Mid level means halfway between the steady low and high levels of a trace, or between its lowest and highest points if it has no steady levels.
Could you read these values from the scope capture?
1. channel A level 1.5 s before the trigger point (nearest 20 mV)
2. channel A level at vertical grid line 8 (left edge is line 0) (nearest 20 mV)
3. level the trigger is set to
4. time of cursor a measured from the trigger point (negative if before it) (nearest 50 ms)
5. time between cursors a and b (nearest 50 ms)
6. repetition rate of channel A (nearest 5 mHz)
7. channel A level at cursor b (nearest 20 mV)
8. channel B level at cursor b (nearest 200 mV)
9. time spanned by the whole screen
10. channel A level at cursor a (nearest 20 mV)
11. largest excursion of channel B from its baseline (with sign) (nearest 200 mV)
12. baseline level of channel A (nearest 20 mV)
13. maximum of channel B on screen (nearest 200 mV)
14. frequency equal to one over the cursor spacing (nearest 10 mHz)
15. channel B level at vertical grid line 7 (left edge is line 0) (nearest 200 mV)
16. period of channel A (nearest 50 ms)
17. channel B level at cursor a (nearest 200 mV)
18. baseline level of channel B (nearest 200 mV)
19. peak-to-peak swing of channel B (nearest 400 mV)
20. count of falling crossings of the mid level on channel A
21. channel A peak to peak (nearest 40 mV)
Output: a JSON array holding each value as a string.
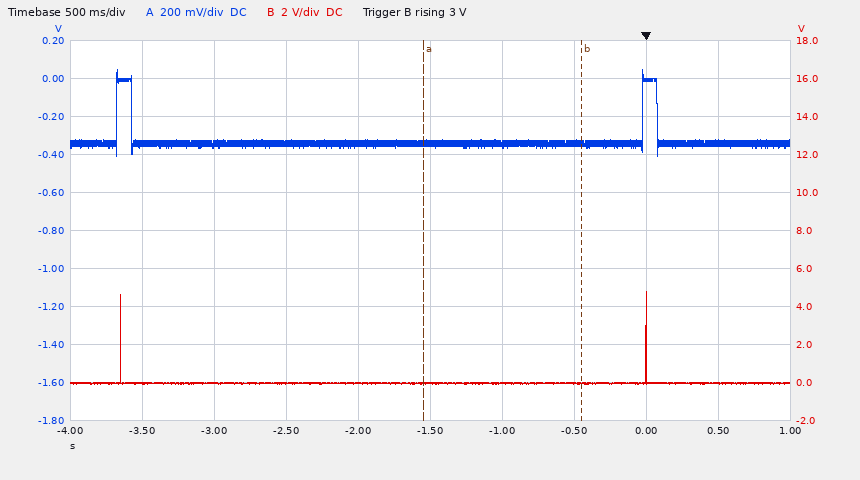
["-340 mV", "0 mV", "3 V", "-1.55 s", "1.10 s", "275 mHz", "-340 mV", "0.0 V", "5 s", "-340 mV", "+4.8 V", "-340 mV", "4.8 V", "910 mHz", "0.0 V", "3.65 s", "0.0 V", "0.0 V", "4.8 V", "2", "440 mV"]
